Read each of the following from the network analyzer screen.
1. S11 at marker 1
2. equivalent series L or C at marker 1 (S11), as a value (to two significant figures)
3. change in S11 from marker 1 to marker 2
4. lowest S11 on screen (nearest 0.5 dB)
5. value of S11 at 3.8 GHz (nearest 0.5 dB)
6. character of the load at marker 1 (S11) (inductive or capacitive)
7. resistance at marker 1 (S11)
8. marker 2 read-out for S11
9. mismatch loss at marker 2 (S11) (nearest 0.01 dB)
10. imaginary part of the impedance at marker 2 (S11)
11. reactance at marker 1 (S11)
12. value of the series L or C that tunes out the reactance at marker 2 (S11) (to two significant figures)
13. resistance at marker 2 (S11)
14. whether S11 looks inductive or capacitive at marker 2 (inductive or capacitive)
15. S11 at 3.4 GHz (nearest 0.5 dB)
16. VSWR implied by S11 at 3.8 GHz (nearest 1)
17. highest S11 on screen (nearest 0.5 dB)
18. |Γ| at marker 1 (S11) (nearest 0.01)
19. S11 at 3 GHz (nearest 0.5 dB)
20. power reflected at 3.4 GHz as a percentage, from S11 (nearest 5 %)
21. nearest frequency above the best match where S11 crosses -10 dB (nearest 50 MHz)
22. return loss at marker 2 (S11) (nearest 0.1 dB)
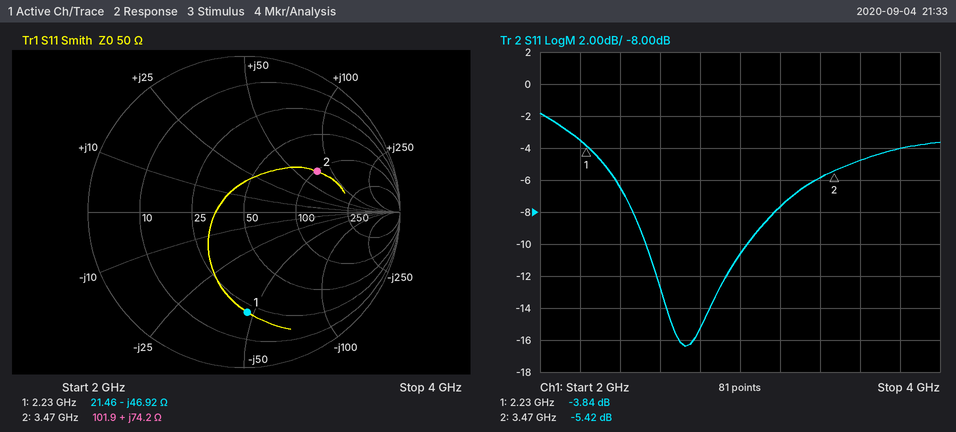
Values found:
-3.84 dB
1.5 pF
-1.58 dB
-16.5 dB
-4.0 dB
capacitive
21.46 Ω
-5.42 dB
1.47 dB
+74.2 Ω
-46.92 Ω
620 fF
101.9 Ω
inductive
-6.0 dB
4
-2.0 dB
0.64
-10.5 dB
25 %
3.05 GHz
5.4 dB
